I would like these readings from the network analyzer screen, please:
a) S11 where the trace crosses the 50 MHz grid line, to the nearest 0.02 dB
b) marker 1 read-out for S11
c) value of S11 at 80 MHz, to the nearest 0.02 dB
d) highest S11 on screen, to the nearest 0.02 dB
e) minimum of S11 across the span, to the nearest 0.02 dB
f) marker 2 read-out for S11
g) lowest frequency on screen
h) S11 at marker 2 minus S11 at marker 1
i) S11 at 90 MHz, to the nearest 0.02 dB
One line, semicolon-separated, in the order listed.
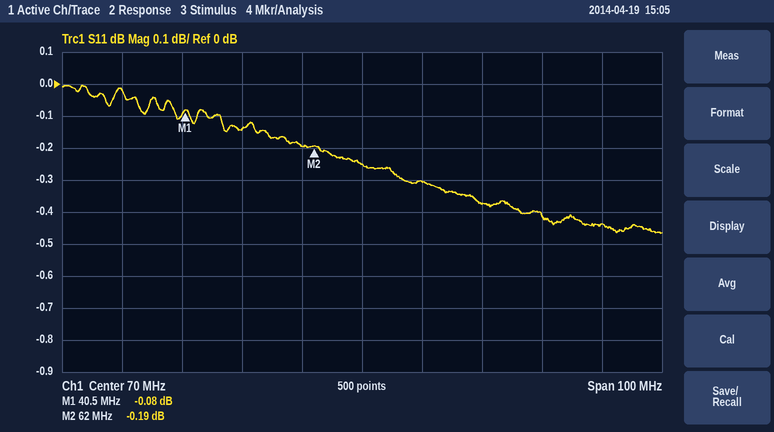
-0.14 dB; -0.08 dB; -0.30 dB; 0.00 dB; -0.46 dB; -0.19 dB; 20 MHz; -0.11 dB; -0.38 dB
